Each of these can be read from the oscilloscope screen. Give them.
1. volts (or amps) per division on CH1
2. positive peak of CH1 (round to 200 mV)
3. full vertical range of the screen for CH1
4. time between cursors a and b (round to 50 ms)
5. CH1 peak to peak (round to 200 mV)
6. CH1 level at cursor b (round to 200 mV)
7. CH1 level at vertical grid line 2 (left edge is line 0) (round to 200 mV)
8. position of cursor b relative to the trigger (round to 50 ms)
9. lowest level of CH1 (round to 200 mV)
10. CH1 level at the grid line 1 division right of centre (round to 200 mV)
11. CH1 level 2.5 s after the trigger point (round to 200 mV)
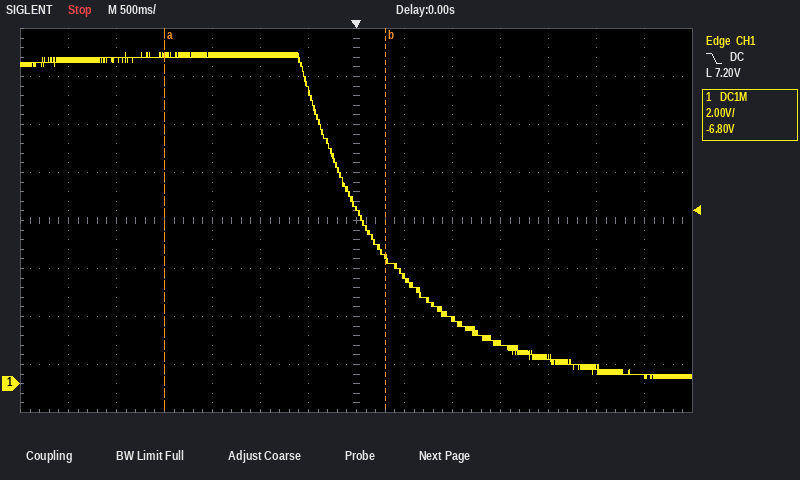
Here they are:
2 V
13.8 V
16 V
2.30 s
13.6 V
5.2 V
13.6 V
+300 ms
200 mV
4.4 V
600 mV
